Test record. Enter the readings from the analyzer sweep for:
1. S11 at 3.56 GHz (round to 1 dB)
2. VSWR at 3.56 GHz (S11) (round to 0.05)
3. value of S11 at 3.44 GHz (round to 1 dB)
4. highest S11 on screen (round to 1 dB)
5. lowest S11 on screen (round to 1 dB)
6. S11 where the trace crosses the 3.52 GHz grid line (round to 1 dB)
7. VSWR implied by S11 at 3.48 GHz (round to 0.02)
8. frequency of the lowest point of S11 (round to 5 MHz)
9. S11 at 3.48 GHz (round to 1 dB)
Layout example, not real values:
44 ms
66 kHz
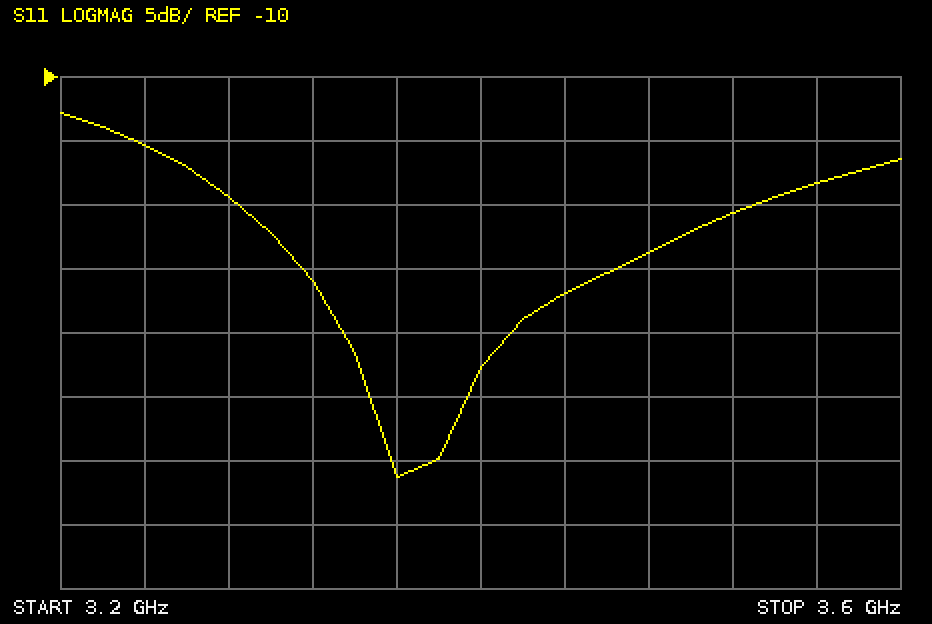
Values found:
-18 dB
1.30
-27 dB
-13 dB
-41 dB
-21 dB
1.14
3.360 GHz
-24 dB
